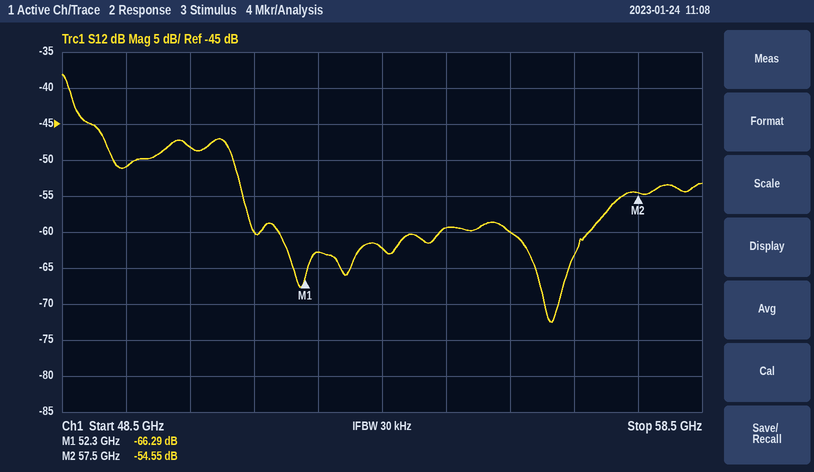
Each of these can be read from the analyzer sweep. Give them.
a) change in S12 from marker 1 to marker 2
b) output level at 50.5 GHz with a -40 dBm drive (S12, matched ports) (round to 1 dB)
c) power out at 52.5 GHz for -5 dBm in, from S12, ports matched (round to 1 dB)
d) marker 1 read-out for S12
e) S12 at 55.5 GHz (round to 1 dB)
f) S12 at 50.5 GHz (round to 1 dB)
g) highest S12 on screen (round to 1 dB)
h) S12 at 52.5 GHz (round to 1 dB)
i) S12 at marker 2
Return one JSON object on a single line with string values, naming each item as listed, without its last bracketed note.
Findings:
{"change in S12 from marker 1 to marker 2": "11.74 dB", "output level at 50.5 GHz with a -40 dBm drive (S12, matched ports)": "-88 dBm", "power out at 52.5 GHz for -5 dBm in, from S12, ports matched": "-68 dBm", "marker 1 read-out for S12": "-66.29 dB", "S12 at 55.5 GHz": "-60 dB", "S12 at 50.5 GHz": "-48 dB", "highest S12 on screen": "-38 dB", "S12 at 52.5 GHz": "-63 dB", "S12 at marker 2": "-54.55 dB"}
